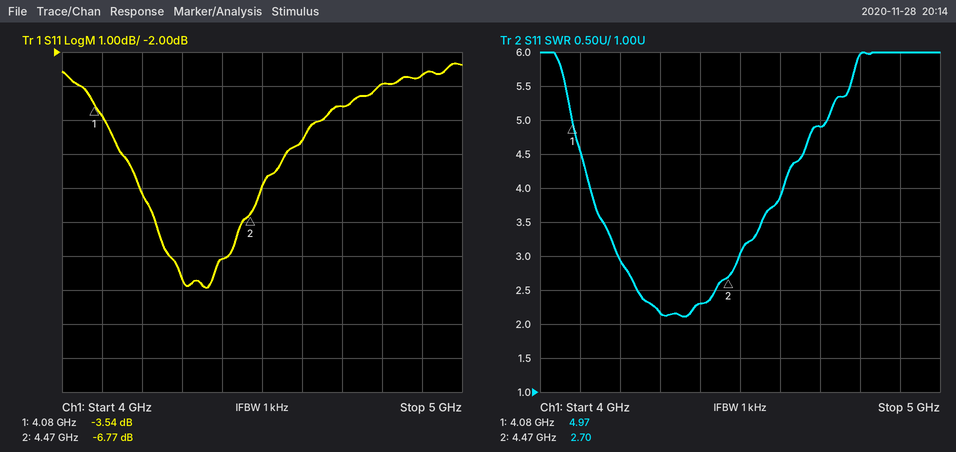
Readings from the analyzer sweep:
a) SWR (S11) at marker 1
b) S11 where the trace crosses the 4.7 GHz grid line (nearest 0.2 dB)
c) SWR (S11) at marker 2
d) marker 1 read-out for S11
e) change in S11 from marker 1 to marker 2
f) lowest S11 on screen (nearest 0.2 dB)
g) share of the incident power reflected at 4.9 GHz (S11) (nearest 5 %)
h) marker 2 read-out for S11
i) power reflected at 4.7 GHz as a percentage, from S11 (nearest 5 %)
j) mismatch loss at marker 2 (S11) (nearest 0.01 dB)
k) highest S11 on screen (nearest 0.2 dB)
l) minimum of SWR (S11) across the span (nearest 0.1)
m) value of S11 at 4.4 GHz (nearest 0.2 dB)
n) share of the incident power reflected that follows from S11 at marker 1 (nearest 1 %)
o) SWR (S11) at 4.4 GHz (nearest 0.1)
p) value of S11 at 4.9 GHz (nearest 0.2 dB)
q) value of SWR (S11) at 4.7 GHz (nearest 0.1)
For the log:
4.97
-3.6 dB
2.70
-3.54 dB
-3.23 dB
-9.0 dB
55 %
-6.77 dB
45 %
1.03 dB
-2.4 dB
2.1
-8.0 dB
44 %
2.3
-2.6 dB
4.9
